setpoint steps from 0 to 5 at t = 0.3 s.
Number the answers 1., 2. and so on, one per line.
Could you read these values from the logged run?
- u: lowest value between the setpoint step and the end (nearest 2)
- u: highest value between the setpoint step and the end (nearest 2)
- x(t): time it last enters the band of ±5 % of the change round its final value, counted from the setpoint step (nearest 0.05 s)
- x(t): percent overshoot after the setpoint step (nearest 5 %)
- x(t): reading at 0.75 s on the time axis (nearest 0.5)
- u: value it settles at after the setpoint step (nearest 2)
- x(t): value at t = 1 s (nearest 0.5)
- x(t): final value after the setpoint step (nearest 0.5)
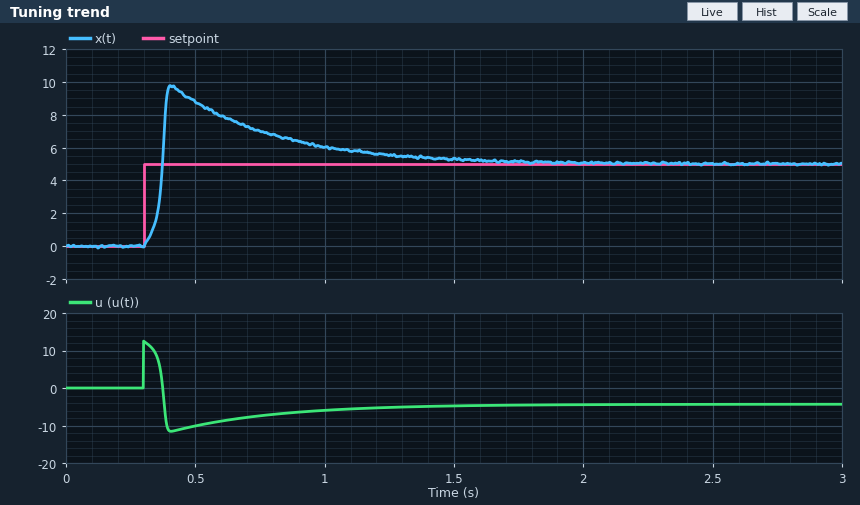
1. -12
2. 12
3. 1.25 s
4. 95 %
5. 7.0
6. -4
7. 6.0
8. 5.0
